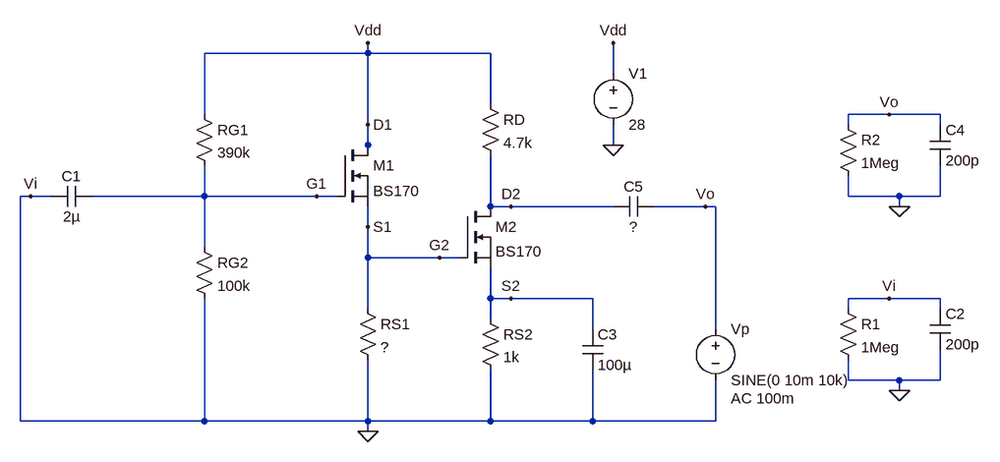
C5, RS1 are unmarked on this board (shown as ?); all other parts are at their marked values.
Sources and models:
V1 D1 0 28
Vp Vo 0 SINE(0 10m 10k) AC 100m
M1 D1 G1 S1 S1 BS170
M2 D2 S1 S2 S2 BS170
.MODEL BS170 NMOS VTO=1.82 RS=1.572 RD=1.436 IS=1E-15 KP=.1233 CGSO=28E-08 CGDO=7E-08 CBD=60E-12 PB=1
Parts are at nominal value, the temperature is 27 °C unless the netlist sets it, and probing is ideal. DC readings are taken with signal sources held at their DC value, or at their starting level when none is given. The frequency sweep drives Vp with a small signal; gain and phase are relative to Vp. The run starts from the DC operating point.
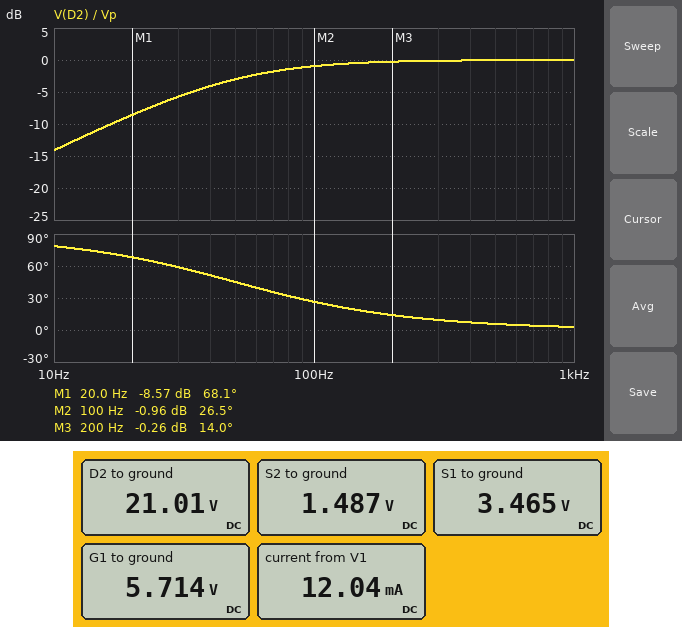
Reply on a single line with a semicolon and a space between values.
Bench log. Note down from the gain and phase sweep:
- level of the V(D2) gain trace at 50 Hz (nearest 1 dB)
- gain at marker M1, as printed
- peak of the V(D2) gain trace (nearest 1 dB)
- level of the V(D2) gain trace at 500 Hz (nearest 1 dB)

-3 dB; -8.57 dB; 0 dB; 0 dB
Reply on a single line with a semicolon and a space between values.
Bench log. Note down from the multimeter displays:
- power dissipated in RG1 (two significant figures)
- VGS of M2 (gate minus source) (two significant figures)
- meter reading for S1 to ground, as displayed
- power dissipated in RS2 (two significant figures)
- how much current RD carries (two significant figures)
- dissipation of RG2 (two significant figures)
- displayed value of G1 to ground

1.3 mW; 2.0 V; 3.465 V; 2.2 mW; 1.5 mA; 330 µW; 5.714 V
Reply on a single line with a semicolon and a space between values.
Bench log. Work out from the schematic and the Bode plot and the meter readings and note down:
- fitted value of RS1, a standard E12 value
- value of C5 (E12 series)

330 Ω; 680 nF
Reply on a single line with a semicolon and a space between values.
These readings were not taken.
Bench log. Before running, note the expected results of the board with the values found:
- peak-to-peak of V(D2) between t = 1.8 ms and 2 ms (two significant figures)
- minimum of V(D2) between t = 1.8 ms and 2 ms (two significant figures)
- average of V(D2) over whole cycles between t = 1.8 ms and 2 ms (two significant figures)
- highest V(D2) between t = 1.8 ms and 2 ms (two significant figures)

20 mV; 21 V; 21 V; 21 V
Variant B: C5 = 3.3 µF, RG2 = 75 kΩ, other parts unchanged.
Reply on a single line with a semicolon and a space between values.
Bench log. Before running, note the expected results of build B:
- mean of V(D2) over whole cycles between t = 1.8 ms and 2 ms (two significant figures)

26 V
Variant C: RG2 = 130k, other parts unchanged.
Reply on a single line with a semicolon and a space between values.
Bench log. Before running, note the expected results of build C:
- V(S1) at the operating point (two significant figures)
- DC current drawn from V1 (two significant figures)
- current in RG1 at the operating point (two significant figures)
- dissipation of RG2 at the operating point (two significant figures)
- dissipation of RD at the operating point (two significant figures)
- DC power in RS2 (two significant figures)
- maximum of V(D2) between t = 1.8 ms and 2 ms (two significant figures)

4.7 V; 17 mA; 54 µA; 380 µW; 33 mW; 7.0 mW; 16 V
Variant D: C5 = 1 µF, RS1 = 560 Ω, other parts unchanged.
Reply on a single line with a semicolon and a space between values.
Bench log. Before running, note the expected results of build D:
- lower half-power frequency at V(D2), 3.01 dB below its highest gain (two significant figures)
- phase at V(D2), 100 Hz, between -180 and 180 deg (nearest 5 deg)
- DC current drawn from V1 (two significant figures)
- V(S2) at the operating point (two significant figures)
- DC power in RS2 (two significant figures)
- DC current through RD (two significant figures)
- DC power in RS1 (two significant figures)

34 Hz; 20 deg; 8.0 mA; 1.6 V; 2.5 mW; 1.6 mA; 23 mW
